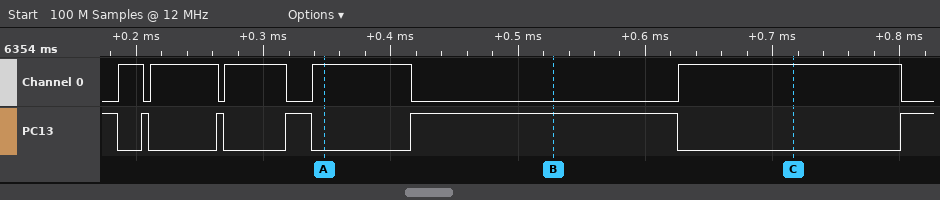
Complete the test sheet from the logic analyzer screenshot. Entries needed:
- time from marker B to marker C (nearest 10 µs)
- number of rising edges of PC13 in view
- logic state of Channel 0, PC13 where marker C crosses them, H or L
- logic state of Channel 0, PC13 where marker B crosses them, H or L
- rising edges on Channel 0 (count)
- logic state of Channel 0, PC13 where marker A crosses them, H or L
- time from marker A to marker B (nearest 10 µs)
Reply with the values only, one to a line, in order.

190 µs
5
Channel 0=H, PC13=L
Channel 0=L, PC13=H
5
Channel 0=H, PC13=L
180 µs
